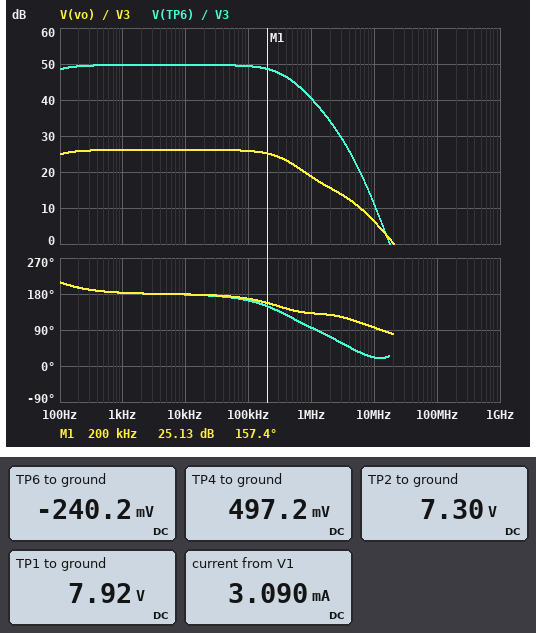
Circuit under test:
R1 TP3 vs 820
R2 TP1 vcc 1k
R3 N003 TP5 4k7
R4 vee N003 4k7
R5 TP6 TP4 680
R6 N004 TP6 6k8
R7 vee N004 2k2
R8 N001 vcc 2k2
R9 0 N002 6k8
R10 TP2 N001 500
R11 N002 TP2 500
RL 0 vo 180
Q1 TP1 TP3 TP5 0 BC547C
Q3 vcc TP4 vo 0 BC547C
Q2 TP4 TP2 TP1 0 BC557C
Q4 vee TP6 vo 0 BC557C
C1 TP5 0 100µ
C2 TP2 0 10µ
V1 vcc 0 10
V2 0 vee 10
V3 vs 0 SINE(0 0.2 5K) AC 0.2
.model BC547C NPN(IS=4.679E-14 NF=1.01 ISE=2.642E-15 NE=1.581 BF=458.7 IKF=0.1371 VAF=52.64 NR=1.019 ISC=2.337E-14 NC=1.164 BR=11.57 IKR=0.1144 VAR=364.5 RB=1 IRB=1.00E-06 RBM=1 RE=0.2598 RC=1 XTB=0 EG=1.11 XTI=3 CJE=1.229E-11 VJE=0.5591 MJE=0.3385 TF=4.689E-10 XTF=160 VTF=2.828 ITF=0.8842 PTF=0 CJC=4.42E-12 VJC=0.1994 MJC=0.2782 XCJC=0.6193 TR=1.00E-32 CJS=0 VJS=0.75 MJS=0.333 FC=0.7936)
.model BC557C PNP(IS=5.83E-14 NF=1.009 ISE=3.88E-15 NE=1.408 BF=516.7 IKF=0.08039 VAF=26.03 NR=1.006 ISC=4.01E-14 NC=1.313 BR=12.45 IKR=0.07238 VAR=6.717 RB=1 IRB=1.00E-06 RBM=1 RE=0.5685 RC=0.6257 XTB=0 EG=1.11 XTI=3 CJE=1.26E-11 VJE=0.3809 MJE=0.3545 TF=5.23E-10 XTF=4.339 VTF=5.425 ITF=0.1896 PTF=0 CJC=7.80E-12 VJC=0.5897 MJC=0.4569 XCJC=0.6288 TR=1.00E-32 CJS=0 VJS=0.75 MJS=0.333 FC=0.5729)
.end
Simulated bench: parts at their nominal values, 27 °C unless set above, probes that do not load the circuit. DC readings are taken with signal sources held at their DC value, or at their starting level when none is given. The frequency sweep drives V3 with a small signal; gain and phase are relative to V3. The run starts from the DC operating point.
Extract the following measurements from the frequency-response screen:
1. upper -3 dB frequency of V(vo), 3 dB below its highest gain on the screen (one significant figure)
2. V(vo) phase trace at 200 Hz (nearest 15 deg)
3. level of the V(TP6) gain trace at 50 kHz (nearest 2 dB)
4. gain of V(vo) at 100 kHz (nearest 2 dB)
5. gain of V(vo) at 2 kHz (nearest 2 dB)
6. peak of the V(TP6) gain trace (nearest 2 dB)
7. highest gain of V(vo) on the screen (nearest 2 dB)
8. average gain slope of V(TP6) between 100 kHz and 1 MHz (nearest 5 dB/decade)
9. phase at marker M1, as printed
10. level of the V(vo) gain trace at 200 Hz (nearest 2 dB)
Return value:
400 kHz
195 deg
50 dB
26 dB
26 dB
50 dB
26 dB
-10 dB/decade
157.4 deg
26 dB
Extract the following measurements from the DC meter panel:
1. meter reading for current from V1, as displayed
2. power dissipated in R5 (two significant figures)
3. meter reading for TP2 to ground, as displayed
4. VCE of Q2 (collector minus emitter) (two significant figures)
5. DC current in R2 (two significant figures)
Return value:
3.090 mA
800 µW
7.30 V
-7.4 V
2.1 mA
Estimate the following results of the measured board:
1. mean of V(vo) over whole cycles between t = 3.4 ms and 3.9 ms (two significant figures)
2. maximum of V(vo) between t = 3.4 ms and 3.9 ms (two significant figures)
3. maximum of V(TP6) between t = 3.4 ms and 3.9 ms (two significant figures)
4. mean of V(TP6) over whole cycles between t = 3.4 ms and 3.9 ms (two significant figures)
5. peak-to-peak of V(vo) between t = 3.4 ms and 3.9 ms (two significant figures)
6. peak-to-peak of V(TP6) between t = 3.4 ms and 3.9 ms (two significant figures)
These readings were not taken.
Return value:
1.8 V
7.2 V
6.7 V
1.2 V
15 V
15 V
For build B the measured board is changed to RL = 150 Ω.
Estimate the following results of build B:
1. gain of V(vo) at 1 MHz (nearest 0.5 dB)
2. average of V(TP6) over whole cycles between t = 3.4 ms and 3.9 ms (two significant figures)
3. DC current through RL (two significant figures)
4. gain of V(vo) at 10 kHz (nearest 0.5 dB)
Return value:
17.0 dB
1.3 V
9.6 µA
24.5 dB
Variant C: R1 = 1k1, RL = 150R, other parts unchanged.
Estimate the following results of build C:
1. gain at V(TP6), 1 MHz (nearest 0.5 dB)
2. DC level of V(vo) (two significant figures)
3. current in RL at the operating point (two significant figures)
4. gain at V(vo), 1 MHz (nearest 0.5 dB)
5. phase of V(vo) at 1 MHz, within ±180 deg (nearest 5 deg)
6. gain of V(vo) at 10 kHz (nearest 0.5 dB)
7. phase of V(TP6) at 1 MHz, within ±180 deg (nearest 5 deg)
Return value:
40.0 dB
1.5 mV
9.8 µA
17.0 dB
125 deg
24.5 dB
90 deg
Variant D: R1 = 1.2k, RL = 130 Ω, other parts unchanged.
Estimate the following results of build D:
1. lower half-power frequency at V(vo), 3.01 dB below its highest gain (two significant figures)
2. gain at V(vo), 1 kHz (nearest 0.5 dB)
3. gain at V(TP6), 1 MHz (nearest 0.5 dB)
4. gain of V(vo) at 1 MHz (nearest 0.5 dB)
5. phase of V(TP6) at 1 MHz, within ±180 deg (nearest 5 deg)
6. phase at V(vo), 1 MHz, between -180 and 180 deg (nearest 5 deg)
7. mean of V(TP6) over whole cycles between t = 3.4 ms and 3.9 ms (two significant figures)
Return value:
55 Hz
23.5 dB
40.0 dB
15.5 dB
90 deg
125 deg
1.3 V
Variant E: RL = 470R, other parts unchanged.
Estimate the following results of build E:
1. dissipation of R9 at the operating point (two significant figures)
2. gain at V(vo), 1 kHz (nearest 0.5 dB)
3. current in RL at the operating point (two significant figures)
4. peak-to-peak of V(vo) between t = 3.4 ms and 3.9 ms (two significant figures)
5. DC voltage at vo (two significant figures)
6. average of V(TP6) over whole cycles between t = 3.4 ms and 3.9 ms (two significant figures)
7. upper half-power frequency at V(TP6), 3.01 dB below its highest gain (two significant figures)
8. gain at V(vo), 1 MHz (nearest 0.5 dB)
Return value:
6.8 mW
33.0 dB
8.7 µA
16 V
4.1 mV
960 mV
390 kHz
26.0 dB
